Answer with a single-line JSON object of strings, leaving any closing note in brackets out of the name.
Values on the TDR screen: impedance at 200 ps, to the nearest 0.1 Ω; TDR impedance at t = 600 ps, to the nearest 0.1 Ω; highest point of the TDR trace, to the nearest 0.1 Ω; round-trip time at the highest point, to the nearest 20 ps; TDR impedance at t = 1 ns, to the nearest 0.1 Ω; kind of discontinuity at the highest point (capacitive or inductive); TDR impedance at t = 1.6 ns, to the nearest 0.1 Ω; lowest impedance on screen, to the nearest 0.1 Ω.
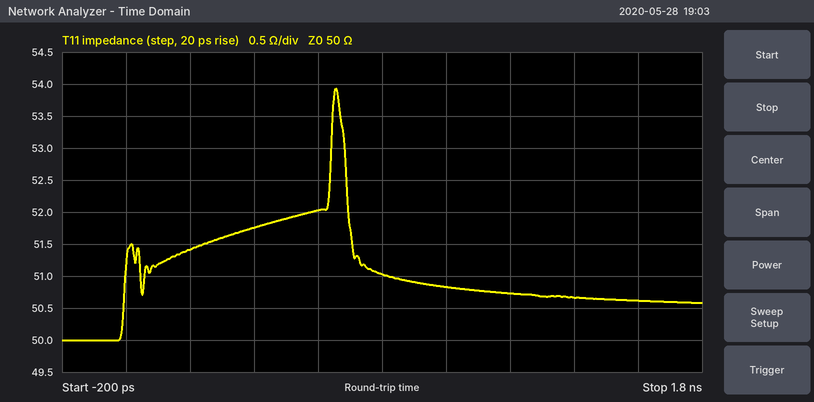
{"impedance at 200 ps, to the nearest 0.1 Ω": "51.4 Ω", "TDR impedance at t = 600 ps, to the nearest 0.1 Ω": "52.0 Ω", "highest point of the TDR trace, to the nearest 0.1 Ω": "53.9 Ω", "round-trip time at the highest point, to the nearest 20 ps": "660 ps", "TDR impedance at t = 1 ns, to the nearest 0.1 Ω": "50.8 Ω", "kind of discontinuity at the highest point": "inductive", "TDR impedance at t = 1.6 ns, to the nearest 0.1 Ω": "50.6 Ω", "lowest impedance on screen, to the nearest 0.1 Ω": "50.0 Ω"}
